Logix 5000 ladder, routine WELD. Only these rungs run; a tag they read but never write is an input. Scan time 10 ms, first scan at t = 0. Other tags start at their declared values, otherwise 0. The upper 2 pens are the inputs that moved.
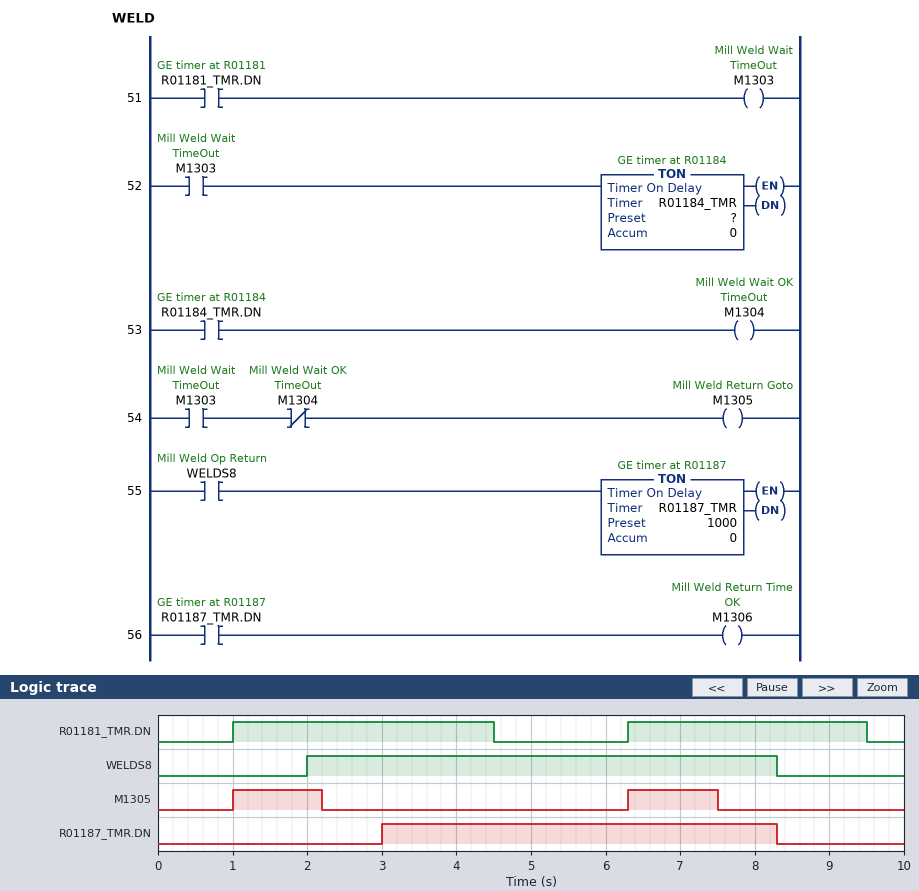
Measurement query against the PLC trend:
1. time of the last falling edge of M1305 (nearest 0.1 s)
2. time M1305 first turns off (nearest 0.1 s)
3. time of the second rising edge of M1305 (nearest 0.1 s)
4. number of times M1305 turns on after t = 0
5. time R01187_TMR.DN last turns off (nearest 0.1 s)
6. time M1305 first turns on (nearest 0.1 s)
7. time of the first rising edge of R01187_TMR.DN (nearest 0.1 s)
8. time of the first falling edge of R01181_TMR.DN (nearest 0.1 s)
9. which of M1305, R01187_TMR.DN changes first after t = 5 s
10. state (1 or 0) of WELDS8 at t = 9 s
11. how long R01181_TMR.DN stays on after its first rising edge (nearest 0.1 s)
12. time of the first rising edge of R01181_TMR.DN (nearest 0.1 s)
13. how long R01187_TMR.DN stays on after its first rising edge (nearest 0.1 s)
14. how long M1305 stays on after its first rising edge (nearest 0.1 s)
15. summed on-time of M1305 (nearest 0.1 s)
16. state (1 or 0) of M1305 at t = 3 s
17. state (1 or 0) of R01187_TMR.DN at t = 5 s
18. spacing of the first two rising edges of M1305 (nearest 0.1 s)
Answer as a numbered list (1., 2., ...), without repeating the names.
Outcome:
1. 7.5 s
2. 2.2 s
3. 6.3 s
4. 2
5. 8.3 s
6. 1.0 s
7. 3.0 s
8. 4.5 s
9. M1305
10. 0
11. 3.5 s
12. 1.0 s
13. 5.3 s
14. 1.2 s
15. 2.4 s
16. 0
17. 1
18. 5.3 s
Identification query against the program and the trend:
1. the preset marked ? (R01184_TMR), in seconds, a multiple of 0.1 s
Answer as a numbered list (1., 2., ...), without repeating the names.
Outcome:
1. 1.2 s
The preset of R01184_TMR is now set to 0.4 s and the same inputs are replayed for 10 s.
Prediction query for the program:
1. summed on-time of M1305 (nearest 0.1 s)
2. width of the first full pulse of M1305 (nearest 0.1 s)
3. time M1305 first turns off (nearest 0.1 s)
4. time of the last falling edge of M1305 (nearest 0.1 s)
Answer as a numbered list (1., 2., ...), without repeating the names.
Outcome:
1. 0.8 s
2. 0.4 s
3. 1.4 s
4. 6.7 s
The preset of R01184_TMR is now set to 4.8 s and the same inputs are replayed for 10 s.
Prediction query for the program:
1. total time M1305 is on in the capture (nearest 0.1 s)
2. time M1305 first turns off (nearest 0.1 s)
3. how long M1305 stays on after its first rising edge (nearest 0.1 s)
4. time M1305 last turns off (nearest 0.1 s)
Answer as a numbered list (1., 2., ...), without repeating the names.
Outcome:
1. 6.7 s
2. 4.5 s
3. 3.5 s
4. 9.5 s
